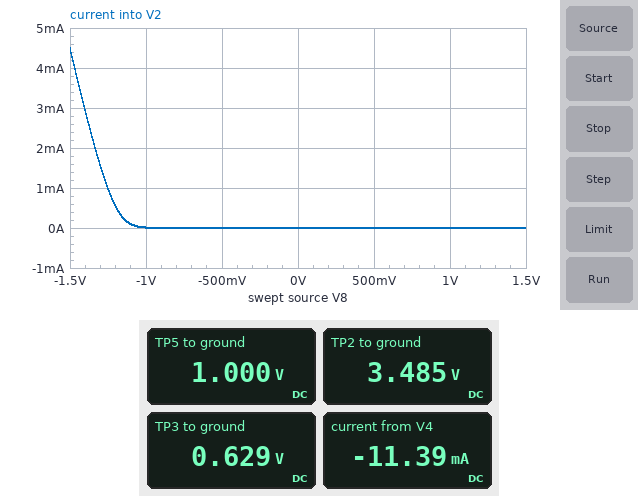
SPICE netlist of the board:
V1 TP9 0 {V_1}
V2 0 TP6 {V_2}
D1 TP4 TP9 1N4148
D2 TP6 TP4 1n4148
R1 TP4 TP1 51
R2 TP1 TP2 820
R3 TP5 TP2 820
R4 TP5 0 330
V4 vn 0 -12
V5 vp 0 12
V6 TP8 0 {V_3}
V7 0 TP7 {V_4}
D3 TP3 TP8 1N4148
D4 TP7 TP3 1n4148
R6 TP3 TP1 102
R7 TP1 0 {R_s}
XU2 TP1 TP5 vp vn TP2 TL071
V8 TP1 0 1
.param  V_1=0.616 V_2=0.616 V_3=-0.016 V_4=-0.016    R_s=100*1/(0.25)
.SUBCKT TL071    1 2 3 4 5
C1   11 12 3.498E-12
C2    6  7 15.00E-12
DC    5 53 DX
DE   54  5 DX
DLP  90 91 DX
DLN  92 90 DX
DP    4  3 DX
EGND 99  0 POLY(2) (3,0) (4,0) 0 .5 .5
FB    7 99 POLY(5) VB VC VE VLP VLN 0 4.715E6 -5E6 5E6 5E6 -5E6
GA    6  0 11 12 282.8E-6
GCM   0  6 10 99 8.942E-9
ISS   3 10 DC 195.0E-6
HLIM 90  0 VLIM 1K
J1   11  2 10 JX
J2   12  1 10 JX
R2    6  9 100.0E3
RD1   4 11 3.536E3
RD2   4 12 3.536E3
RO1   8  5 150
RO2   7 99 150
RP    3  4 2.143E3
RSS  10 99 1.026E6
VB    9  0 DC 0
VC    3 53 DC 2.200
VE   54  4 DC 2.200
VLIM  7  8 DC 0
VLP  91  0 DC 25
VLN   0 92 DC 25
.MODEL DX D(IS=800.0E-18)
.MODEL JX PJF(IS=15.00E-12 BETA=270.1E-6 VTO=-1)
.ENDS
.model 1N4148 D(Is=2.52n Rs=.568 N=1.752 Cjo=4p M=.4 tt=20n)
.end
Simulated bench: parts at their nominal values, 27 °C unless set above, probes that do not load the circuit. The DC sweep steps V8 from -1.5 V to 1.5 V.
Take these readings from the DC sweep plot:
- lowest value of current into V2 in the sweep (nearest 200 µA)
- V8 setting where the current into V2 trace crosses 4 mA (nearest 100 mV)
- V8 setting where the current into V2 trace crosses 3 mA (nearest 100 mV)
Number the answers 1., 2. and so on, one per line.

1. 0 A
2. -1.5 V
3. -1.4 V
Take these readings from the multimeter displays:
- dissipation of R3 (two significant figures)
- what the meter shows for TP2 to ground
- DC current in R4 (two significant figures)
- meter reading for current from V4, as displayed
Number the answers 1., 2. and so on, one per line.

1. 7.5 mW
2. 3.485 V
3. 3.0 mA
4. -11.39 mA
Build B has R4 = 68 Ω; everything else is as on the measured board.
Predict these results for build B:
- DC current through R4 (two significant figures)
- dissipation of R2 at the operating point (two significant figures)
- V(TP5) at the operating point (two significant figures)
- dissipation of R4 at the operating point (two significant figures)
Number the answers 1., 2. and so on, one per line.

1. 12 mA
2. 110 mW
3. 800 mV
4. 9.4 mW
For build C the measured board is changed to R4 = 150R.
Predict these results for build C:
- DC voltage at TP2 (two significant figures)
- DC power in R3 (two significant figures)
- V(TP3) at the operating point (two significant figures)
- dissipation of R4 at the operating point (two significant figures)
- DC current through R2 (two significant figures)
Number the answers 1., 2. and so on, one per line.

1. 6.5 V
2. 36 mW
3. 630 mV
4. 6.7 mW
5. 6.7 mA
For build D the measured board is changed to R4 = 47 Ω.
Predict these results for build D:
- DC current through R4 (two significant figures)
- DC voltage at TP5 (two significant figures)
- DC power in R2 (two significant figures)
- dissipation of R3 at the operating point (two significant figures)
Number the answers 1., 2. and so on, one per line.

1. 12 mA
2. 570 mV
3. 110 mW
4. 120 mW
